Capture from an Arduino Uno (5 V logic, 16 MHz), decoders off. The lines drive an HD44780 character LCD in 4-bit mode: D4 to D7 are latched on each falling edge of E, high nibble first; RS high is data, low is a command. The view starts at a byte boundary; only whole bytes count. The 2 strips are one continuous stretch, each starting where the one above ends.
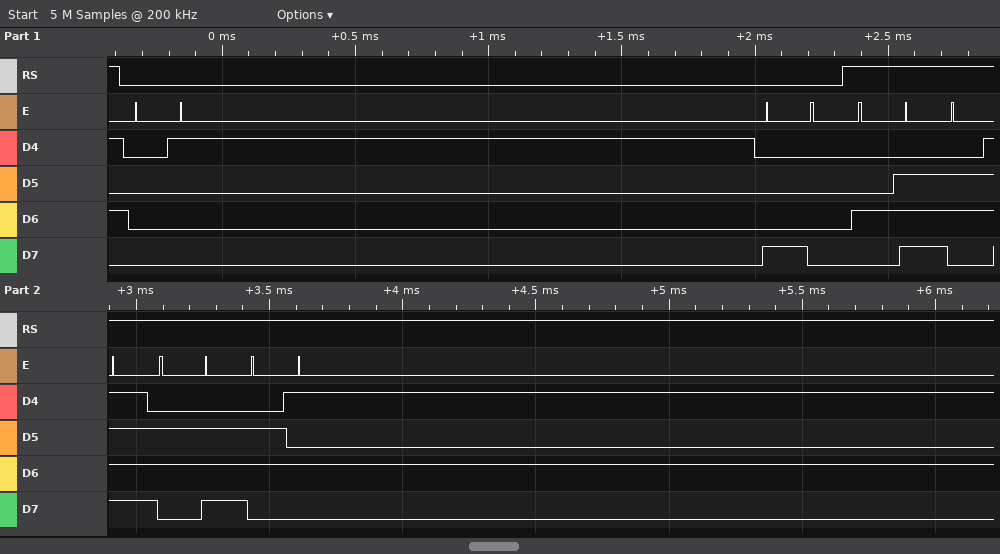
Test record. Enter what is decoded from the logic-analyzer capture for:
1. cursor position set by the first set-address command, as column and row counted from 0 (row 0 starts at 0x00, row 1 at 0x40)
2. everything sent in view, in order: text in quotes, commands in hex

column 0, row 0
0x01 0x80 "None"
